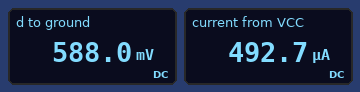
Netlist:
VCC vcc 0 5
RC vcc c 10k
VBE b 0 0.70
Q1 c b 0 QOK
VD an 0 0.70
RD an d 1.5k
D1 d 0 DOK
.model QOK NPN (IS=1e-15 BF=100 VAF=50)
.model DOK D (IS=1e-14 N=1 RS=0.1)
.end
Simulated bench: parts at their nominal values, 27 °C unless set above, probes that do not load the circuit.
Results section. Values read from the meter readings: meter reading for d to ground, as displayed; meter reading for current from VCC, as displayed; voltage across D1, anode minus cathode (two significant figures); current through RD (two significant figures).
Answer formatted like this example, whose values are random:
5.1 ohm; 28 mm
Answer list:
588.0 mV; 492.7 µA; 590 mV; 75 µA
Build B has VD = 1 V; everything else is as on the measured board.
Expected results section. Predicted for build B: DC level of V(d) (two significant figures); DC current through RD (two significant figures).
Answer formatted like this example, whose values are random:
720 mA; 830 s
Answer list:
620 mV; 250 µA
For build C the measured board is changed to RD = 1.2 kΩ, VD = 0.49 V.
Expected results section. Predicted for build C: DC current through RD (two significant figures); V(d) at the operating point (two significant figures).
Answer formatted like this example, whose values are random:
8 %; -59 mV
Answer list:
1.6 µA; 490 mV
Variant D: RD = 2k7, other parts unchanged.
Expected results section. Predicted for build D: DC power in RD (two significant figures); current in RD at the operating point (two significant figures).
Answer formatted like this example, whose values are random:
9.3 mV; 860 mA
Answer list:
5.7 µW; 46 µA
